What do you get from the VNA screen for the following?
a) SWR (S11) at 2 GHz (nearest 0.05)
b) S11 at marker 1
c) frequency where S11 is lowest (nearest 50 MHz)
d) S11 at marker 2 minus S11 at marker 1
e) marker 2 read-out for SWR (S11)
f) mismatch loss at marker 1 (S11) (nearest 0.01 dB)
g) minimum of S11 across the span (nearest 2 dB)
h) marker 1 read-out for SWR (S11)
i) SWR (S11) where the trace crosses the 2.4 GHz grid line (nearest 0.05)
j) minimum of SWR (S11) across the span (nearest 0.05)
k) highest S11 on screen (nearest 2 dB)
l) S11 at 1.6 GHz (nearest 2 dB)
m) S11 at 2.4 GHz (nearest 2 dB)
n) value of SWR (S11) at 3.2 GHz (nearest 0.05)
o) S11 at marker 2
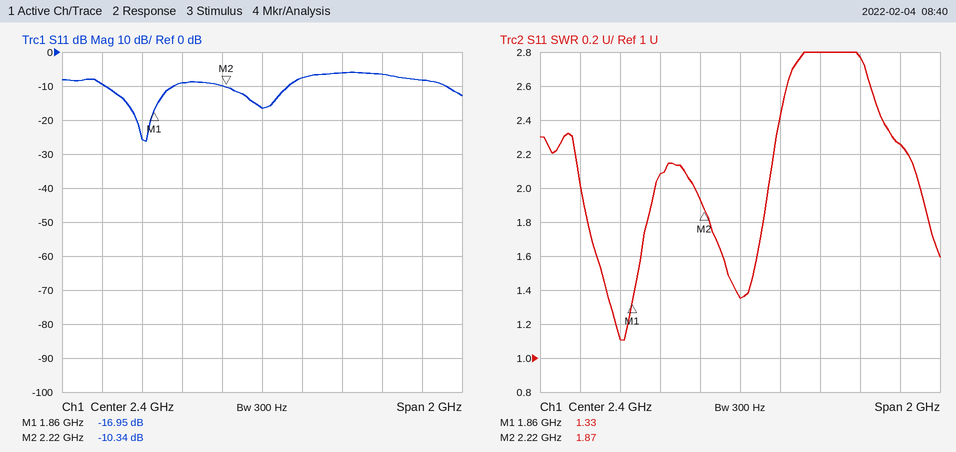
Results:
2.10
-16.95 dB
1.80 GHz
6.61 dB
1.87
0.09 dB
-26 dB
1.33
1.35
1.10
-6 dB
-10 dB
-16 dB
2.25
-10.34 dB
